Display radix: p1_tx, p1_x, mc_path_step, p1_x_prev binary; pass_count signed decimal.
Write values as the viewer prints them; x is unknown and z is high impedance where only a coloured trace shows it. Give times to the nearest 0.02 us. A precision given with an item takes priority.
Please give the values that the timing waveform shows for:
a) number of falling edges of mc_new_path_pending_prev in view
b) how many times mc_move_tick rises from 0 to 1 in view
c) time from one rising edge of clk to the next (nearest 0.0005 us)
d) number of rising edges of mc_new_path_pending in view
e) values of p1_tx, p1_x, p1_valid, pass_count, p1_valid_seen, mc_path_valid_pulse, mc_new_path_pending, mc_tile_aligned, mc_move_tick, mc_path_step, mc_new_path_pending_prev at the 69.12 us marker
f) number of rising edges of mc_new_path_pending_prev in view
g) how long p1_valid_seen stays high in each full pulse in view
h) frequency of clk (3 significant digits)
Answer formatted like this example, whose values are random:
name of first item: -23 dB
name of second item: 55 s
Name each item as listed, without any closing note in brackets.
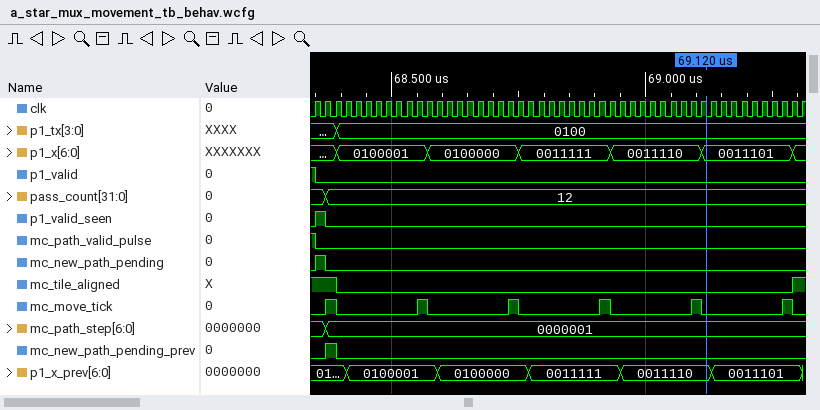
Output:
number of falling edges of mc_new_path_pending_prev in view: 1
how many times mc_move_tick rises from 0 to 1 in view: 6
time from one rising edge of clk to the next: 0.02 us
number of rising edges of mc_new_path_pending in view: 1
values of p1_tx, p1_x, p1_valid, pass_count, p1_valid_seen, mc_path_valid_pulse, mc_new_path_pending, mc_tile_aligned, mc_move_tick, mc_path_step, mc_new_path_pending_prev at the 69.12 us marker: p1_tx=0100, p1_x=0011101, p1_valid=0, pass_count=12, p1_valid_seen=0, mc_path_valid_pulse=0, mc_new_path_pending=0, mc_tile_aligned=0, mc_move_tick=0, mc_path_step=0000001, mc_new_path_pending_prev=0
number of rising edges of mc_new_path_pending_prev in view: 1
how long p1_valid_seen stays high in each full pulse in view: 0.02 us
frequency of clk: 50.0 MHz
